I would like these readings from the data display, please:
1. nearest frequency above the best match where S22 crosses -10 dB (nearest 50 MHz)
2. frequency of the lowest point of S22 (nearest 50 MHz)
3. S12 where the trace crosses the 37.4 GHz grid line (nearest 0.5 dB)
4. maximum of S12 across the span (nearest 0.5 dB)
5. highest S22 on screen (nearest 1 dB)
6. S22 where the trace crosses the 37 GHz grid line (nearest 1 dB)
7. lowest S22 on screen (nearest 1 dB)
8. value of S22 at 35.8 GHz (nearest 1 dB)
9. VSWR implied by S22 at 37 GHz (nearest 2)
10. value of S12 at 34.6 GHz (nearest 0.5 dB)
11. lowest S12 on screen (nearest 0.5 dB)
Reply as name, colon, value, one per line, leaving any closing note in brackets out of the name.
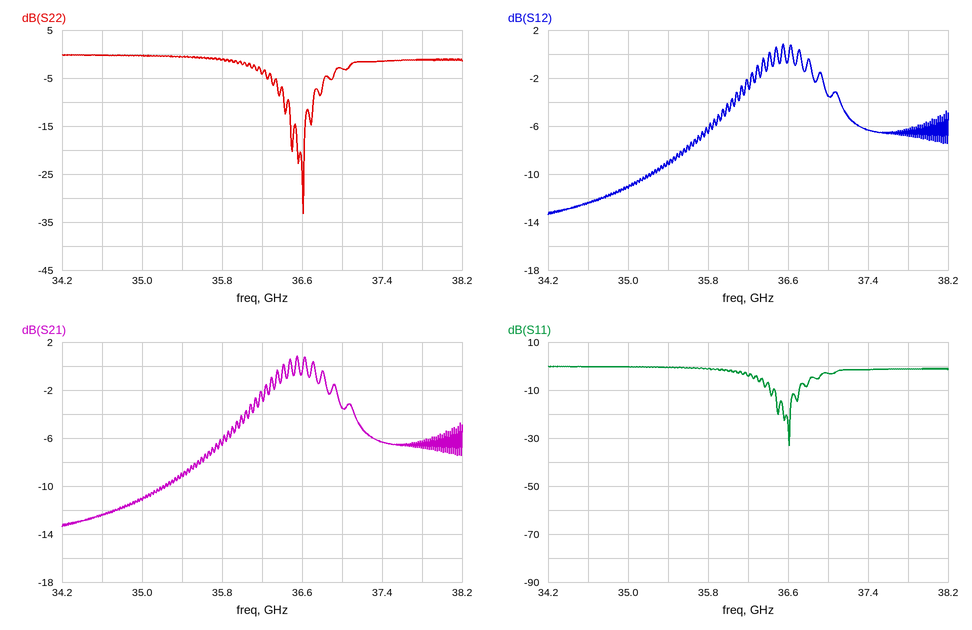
nearest frequency above the best match where S22 crosses -10 dB: 36.70 GHz
frequency of the lowest point of S22: 36.60 GHz
S12 where the trace crosses the 37.4 GHz grid line: -6.5 dB
maximum of S12 across the span: 1.0 dB
highest S22 on screen: 0 dB
S22 where the trace crosses the 37 GHz grid line: -3 dB
lowest S22 on screen: -33 dB
value of S22 at 35.8 GHz: -1 dB
VSWR implied by S22 at 37 GHz: 6
value of S12 at 34.6 GHz: -12.5 dB
lowest S12 on screen: -13.5 dB
